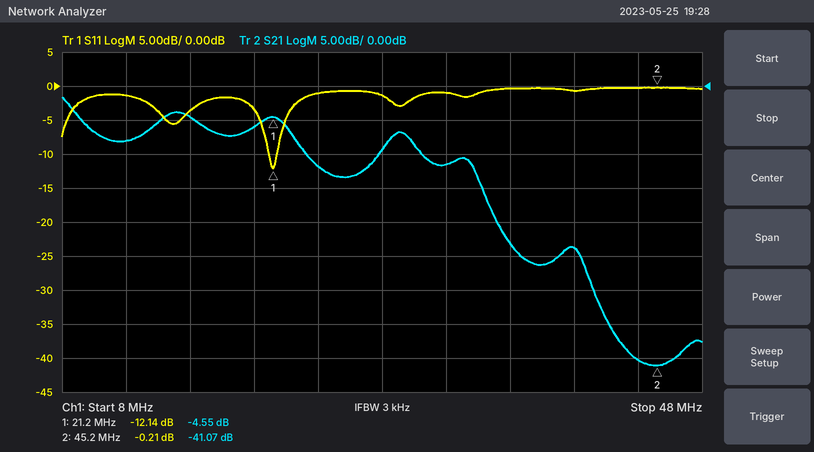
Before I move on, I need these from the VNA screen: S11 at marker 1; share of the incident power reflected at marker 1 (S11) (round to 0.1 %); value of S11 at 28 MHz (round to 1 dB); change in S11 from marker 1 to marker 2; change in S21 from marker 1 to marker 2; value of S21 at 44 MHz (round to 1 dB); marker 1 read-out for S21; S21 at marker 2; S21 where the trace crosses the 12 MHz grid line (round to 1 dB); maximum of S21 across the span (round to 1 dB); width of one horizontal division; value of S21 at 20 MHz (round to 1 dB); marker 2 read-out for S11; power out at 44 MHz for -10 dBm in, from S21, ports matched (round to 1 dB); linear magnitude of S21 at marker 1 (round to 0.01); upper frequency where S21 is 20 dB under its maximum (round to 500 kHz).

-12.14 dB
6.1 %
-1 dB
11.93 dB
-36.52 dB
-40 dB
-4.55 dB
-41.07 dB
-8 dB
-2 dB
4 MHz
-6 dB
-0.21 dB
-50 dBm
0.59
35.5 MHz
